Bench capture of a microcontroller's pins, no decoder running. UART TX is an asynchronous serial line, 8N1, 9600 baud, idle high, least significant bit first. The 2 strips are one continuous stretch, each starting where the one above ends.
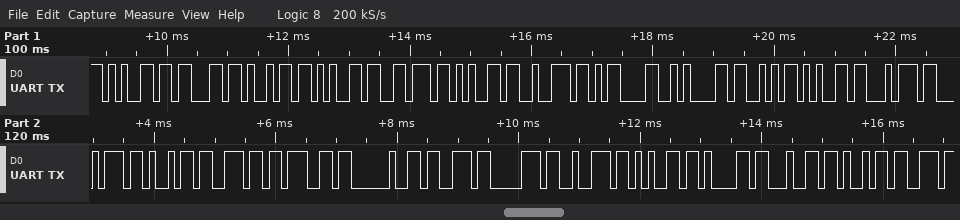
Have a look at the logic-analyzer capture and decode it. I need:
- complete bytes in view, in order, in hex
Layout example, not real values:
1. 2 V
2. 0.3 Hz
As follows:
1. 0x65 0x63 0x69 0x65 0x76 0x65 0x72 0x0D 0x0A 0x53 0x65 0x74 0x74 0x69 0x6E 0x67 0x20 0x73 0x70 0x72 0x65 0x61 0x64 0x69
